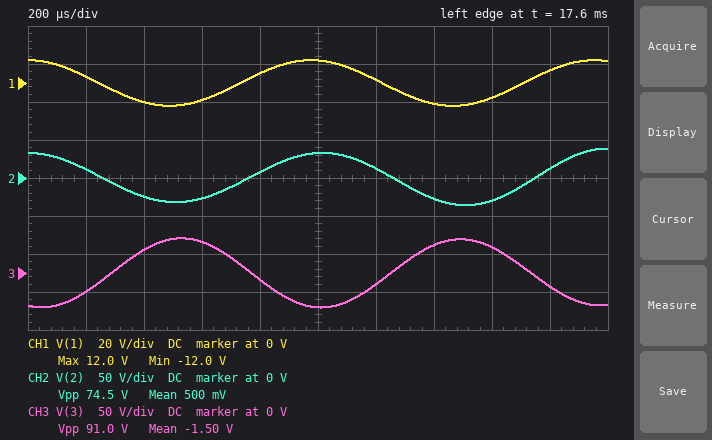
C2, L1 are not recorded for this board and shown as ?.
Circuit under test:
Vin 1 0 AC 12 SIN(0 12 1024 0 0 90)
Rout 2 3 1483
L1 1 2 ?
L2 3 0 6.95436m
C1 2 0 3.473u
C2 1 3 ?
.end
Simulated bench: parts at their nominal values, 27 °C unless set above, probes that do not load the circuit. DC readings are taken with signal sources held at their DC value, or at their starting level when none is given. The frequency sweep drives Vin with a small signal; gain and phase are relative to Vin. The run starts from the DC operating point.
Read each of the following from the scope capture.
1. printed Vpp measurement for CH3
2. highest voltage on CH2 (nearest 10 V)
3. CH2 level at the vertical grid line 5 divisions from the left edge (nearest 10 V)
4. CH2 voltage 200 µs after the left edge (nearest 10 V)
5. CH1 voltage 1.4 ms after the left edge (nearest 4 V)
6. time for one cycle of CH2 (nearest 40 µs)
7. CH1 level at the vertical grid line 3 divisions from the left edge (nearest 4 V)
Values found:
91.0 V
40 V
30 V
10 V
-12 V
1.00 ms
-8 V
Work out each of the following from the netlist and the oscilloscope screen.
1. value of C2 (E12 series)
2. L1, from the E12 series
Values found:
2.7 µF
4.7 mH
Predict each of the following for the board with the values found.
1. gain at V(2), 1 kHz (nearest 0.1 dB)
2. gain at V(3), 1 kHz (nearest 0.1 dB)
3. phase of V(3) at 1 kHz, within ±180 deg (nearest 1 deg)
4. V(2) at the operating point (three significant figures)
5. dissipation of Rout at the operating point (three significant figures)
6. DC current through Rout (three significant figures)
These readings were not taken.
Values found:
8.9 dB
9.0 dB
167 deg
12.0 V
97.1 mW
8.09 mA
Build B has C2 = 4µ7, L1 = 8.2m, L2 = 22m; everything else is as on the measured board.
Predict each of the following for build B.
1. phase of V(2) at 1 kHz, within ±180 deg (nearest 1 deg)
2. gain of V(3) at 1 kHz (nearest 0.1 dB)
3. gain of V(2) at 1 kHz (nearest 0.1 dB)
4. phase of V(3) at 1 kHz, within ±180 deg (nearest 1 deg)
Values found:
-162 deg
2.1 dB
17.7 dB
12 deg
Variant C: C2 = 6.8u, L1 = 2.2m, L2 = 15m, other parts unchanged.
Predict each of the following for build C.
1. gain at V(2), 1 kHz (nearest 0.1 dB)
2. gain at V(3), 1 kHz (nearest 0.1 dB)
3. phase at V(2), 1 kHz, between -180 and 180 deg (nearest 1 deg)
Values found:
3.1 dB
2.5 dB
0 deg
